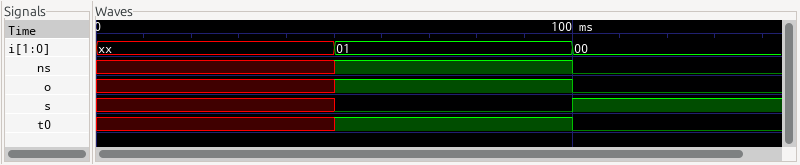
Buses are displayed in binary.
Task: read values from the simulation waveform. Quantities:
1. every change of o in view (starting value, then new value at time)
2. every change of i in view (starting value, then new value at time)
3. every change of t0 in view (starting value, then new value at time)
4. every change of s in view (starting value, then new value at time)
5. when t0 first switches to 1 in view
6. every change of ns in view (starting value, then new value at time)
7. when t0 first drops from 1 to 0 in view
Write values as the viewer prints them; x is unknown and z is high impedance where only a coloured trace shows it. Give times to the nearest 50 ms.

x, 1 at 50 ms, 0 at 100 ms
xx, 01 at 50 ms, 00 at 100 ms
x, 1 at 50 ms, 0 at 100 ms
x, 0 at 50 ms, 1 at 100 ms
50 ms
x, 1 at 50 ms, 0 at 100 ms
100 ms
